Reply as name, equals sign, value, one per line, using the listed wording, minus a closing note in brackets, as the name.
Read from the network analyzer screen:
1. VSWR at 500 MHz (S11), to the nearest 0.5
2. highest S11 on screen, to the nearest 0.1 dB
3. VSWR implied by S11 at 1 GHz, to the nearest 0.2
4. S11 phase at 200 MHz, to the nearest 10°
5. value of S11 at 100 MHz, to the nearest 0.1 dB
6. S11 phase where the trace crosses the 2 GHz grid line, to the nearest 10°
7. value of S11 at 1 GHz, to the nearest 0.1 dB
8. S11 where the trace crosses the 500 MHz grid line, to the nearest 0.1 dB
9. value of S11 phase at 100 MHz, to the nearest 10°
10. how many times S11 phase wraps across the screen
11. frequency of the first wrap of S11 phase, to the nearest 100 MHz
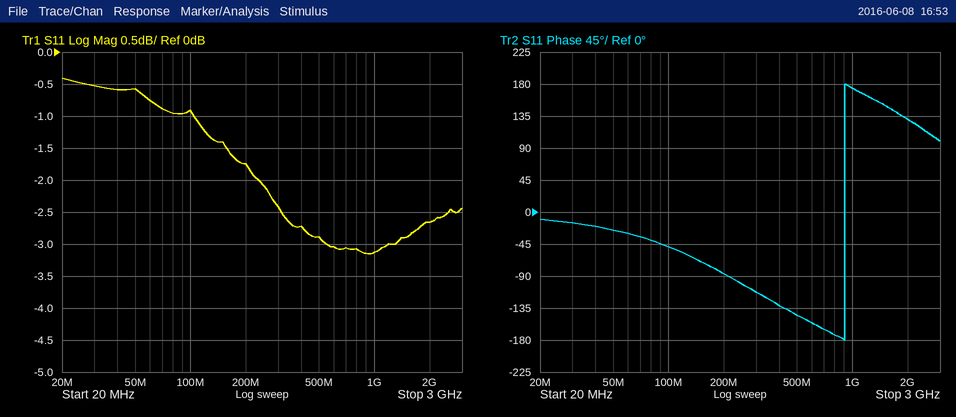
VSWR at 500 MHz (S11), to the nearest 0.5 = 6.0
highest S11 on screen, to the nearest 0.1 dB = -0.4 dB
VSWR implied by S11 at 1 GHz, to the nearest 0.2 = 5.6
S11 phase at 200 MHz, to the nearest 10° = -90°
value of S11 at 100 MHz, to the nearest 0.1 dB = -0.9 dB
S11 phase where the trace crosses the 2 GHz grid line, to the nearest 10° = 130°
value of S11 at 1 GHz, to the nearest 0.1 dB = -3.1 dB
S11 where the trace crosses the 500 MHz grid line, to the nearest 0.1 dB = -2.9 dB
value of S11 phase at 100 MHz, to the nearest 10° = -50°
how many times S11 phase wraps across the screen = 1
frequency of the first wrap of S11 phase, to the nearest 100 MHz = 900 MHz
